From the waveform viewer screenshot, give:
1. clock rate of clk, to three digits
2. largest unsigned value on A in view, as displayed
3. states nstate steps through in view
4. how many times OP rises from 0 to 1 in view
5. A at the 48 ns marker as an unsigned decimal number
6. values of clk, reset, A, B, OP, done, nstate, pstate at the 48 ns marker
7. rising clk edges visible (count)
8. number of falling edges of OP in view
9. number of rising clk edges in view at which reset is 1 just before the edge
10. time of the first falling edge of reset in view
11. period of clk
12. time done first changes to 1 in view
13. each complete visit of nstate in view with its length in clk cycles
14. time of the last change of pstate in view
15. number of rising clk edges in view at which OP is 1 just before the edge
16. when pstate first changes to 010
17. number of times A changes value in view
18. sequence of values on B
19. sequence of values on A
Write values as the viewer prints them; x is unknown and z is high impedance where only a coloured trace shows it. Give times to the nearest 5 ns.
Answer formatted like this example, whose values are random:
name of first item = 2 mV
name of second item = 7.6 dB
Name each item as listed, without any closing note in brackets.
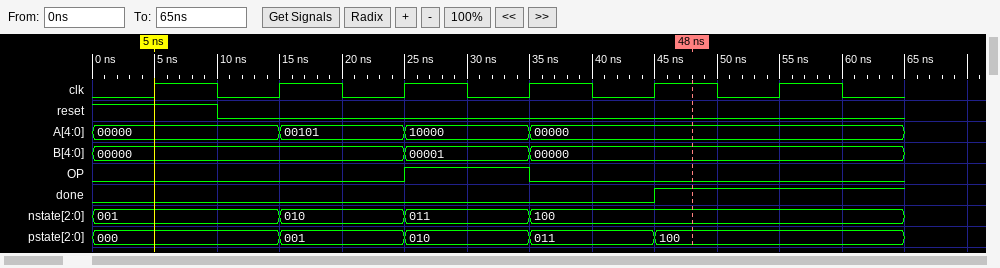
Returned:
clock rate of clk, to three digits = 100 MHz
largest unsigned value on A in view, as displayed = 10000
states nstate steps through in view = 001, 010, 011, 100
how many times OP rises from 0 to 1 in view = 1
A at the 48 ns marker as an unsigned decimal number = 0
values of clk, reset, A, B, OP, done, nstate, pstate at the 48 ns marker = clk=1, reset=0, A=00000, B=00000, OP=0, done=1, nstate=100, pstate=100
rising clk edges visible = 6
number of falling edges of OP in view = 1
number of rising clk edges in view at which reset is 1 just before the edge = 1
time of the first falling edge of reset in view = 10 ns
period of clk = 10 ns
time done first changes to 1 in view = 45 ns
each complete visit of nstate in view with its length in clk cycles = 010: 1, 011: 1
time of the last change of pstate in view = 45 ns
number of rising clk edges in view at which OP is 1 just before the edge = 1
when pstate first changes to 010 = 25 ns
number of times A changes value in view = 3
sequence of values on B = 00000, 00001, 00000
sequence of values on A = 00000, 00101, 10000, 00000
